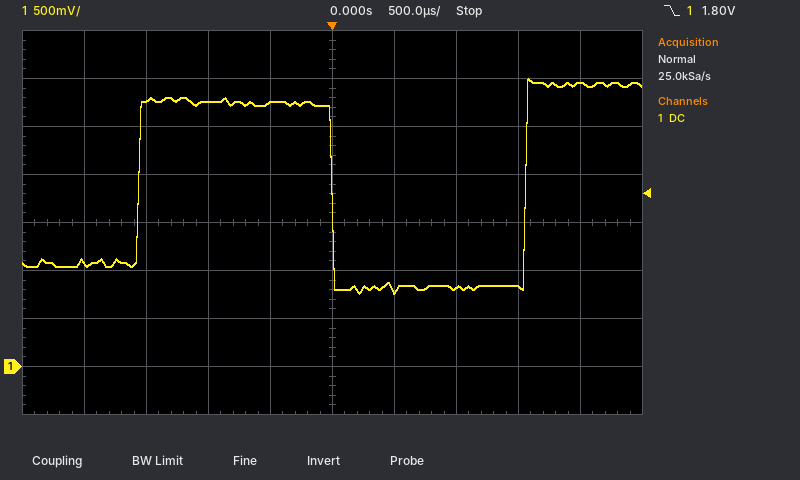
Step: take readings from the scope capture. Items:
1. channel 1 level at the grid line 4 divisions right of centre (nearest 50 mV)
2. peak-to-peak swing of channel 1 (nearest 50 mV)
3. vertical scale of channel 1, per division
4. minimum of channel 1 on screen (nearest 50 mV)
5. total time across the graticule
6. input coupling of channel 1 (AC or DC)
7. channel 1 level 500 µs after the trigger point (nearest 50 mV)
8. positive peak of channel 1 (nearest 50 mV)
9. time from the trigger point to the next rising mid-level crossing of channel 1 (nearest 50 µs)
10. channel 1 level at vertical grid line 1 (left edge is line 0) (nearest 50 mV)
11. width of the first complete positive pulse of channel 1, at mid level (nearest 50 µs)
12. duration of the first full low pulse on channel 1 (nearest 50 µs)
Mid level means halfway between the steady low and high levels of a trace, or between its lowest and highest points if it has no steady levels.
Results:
2.95 V
2.25 V
500 mV
750 mV
5 ms
DC
800 mV
3.00 V
1.55 ms
1.10 V
1.55 ms
1.55 ms
